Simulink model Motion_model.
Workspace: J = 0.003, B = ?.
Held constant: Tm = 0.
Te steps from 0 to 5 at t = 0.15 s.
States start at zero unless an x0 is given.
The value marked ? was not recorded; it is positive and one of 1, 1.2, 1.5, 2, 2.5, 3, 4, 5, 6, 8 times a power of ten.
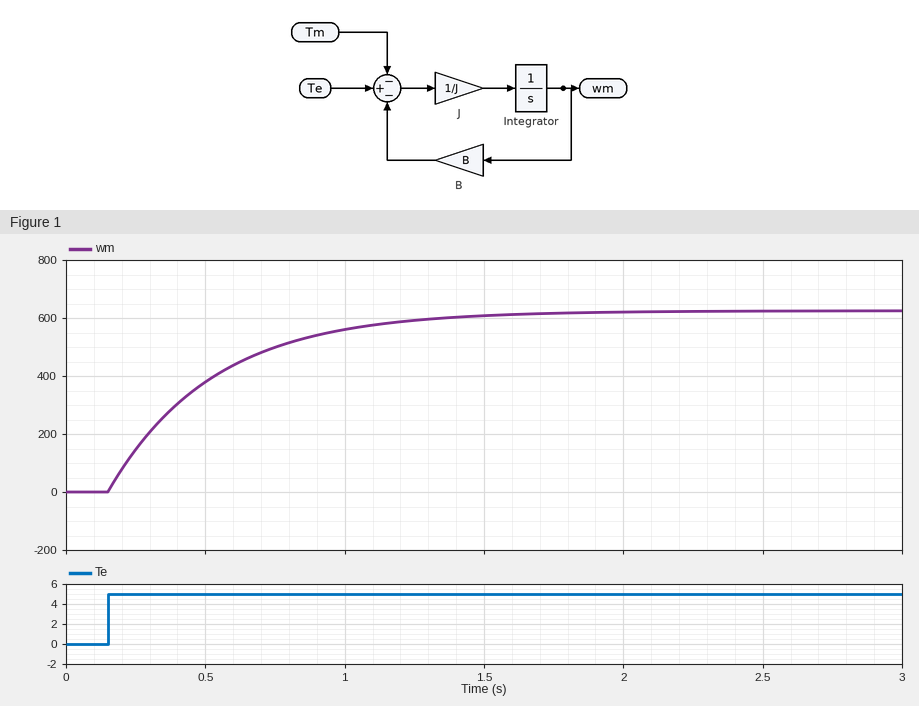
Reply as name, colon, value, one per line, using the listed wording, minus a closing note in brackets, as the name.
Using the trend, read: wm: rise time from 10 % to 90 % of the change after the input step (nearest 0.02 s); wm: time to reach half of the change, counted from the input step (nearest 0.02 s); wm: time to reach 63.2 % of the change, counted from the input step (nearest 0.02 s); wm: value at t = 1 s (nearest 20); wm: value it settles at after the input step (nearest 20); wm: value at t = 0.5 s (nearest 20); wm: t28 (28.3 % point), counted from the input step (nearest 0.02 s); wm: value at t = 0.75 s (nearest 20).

wm: rise time from 10 % to 90 % of the change after the input step: 0.82 s
wm: time to reach half of the change, counted from the input step: 0.26 s
wm: time to reach 63.2 % of the change, counted from the input step: 0.38 s
wm: value at t = 1 s: 560
wm: value it settles at after the input step: 620
wm: value at t = 0.5 s: 380
wm: t28 (28.3 % point), counted from the input step: 0.12 s
wm: value at t = 0.75 s: 500
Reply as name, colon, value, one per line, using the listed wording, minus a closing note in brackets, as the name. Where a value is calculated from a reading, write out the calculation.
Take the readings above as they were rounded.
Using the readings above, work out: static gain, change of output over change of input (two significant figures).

static gain, change of output over change of input: (620 - 0) / (5 - 0) = 120
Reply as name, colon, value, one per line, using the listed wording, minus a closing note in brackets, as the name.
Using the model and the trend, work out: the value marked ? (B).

the value marked ?: 0.008
